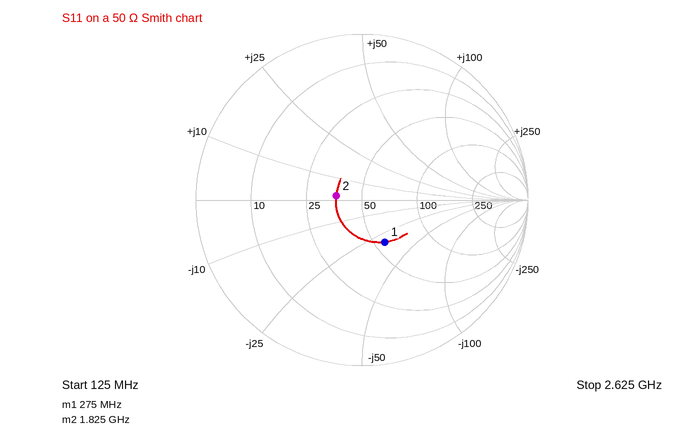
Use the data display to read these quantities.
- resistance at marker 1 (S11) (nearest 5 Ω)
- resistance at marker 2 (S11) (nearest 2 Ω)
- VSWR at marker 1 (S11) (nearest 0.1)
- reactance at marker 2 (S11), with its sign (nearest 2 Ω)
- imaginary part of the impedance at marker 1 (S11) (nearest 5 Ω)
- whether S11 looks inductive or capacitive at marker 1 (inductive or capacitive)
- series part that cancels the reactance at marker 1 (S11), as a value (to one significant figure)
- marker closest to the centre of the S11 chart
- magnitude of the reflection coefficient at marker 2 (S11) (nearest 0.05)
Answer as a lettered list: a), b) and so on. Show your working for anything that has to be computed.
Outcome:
a) 55 Ω
b) 36 Ω
c) 1.8
d) +2 Ω
e) -30 Ω
f) capacitive
g) L = 30 Ω/(2π × 275 MHz) ≈ 17.4 nH, so 20 nH to one significant figure
h) marker 2
i) 0.15
